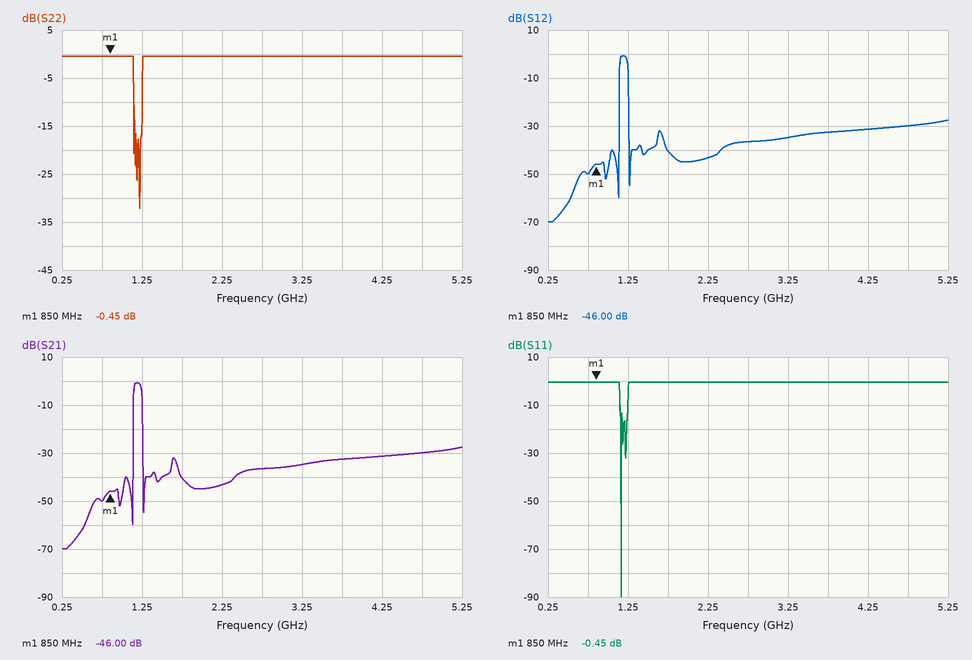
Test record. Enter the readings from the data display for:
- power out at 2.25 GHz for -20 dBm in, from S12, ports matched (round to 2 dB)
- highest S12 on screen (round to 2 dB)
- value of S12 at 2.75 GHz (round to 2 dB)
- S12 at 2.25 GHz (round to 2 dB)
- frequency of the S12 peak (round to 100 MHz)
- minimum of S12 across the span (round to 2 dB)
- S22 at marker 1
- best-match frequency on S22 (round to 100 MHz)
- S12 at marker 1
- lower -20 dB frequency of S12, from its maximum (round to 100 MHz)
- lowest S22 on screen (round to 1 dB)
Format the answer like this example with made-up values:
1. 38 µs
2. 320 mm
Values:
1. -64 dBm
2. 0 dB
3. -36 dB
4. -44 dB
5. 1.2 GHz
6. -70 dB
7. -0.45 dB
8. 1.2 GHz
9. -46.00 dB
10. 1.1 GHz
11. -32 dB
